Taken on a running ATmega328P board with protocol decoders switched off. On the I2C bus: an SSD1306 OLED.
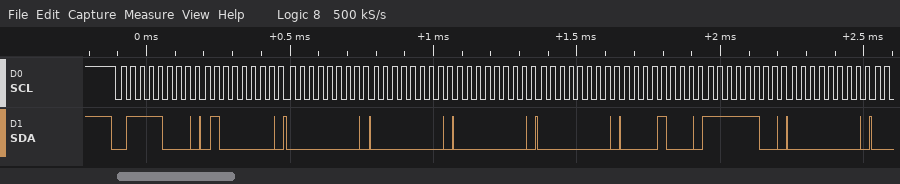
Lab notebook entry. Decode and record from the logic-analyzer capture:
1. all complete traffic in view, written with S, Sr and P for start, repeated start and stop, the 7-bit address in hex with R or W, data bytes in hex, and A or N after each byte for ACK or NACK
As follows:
S 3CW A 40 A 00 A 00 A 00 A 00 A 08 A FC A 00 A
